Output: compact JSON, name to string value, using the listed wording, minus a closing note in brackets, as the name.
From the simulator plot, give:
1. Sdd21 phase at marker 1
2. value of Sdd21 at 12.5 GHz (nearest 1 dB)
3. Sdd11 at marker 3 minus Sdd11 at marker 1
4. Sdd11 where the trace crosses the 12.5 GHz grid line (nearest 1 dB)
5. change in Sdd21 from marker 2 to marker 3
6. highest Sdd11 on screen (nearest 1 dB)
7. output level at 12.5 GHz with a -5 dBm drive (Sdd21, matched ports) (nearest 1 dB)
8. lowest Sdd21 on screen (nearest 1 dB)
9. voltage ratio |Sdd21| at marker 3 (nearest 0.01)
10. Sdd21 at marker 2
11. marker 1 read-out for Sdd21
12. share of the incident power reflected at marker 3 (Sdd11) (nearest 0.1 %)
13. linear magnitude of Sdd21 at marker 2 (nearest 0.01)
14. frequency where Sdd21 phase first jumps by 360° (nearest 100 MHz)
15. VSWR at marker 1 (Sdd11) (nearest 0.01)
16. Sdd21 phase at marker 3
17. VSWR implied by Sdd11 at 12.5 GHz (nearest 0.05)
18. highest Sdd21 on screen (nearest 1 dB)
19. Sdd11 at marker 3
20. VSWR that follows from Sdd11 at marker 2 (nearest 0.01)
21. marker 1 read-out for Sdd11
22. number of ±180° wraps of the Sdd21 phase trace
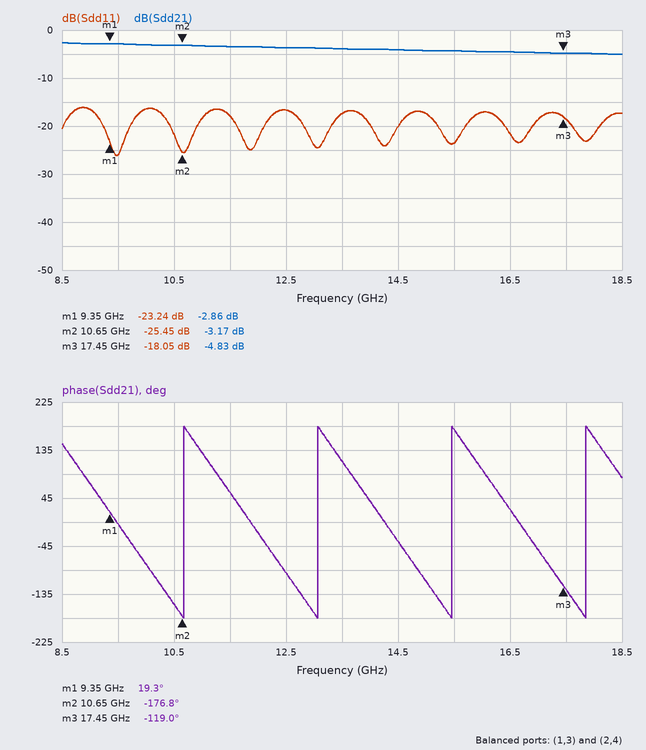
{"Sdd21 phase at marker 1": "19.3°", "value of Sdd21 at 12.5 GHz": "-4 dB", "Sdd11 at marker 3 minus Sdd11 at marker 1": "5.19 dB", "Sdd11 where the trace crosses the 12.5 GHz grid line": "-17 dB", "change in Sdd21 from marker 2 to marker 3": "-1.66 dB", "highest Sdd11 on screen": "-16 dB", "output level at 12.5 GHz with a -5 dBm drive (Sdd21, matched ports)": "-9 dBm", "lowest Sdd21 on screen": "-5 dB", "voltage ratio |Sdd21| at marker 3": "0.57", "Sdd21 at marker 2": "-3.17 dB", "marker 1 read-out for Sdd21": "-2.86 dB", "share of the incident power reflected at marker 3 (Sdd11)": "1.6 %", "linear magnitude of Sdd21 at marker 2": "0.69", "frequency where Sdd21 phase first jumps by 360°": "10.7 GHz", "VSWR at marker 1 (Sdd11)": "1.15", "Sdd21 phase at marker 3": "-119.0°", "VSWR implied by Sdd11 at 12.5 GHz": "1.35", "highest Sdd21 on screen": "-3 dB", "Sdd11 at marker 3": "-18.05 dB", "VSWR that follows from Sdd11 at marker 2": "1.11", "marker 1 read-out for Sdd11": "-23.24 dB", "number of ±180° wraps of the Sdd21 phase trace": "4"}
